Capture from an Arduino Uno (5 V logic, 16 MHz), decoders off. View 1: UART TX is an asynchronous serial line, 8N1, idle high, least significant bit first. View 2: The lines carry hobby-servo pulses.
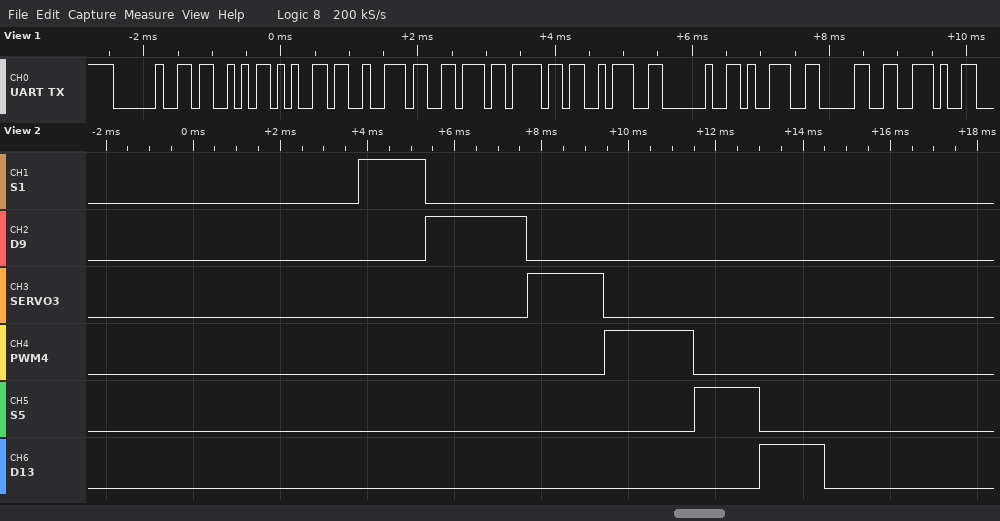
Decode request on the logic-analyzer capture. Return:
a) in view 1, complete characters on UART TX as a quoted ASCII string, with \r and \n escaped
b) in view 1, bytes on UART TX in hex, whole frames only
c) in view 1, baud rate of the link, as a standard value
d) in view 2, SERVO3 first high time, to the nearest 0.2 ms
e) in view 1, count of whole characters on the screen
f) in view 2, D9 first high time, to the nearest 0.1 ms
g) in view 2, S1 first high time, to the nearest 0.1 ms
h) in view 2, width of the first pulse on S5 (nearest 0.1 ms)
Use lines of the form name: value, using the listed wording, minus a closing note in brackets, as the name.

in view 1, complete characters on UART TX as a quoted ASCII string, with \r and \n escaped: " Servo: 90."
in view 1, bytes on UART TX in hex, whole frames only: 20 53 65 72 76 6F 3A 20 39 30 2E
in view 1, baud rate of the link, as a standard value: 9600 baud
in view 2, SERVO3 first high time, to the nearest 0.2 ms: 1.8 ms
in view 1, count of whole characters on the screen: 11
in view 2, D9 first high time, to the nearest 0.1 ms: 2.3 ms
in view 2, S1 first high time, to the nearest 0.1 ms: 1.5 ms
in view 2, width of the first pulse on S5: 1.5 ms
